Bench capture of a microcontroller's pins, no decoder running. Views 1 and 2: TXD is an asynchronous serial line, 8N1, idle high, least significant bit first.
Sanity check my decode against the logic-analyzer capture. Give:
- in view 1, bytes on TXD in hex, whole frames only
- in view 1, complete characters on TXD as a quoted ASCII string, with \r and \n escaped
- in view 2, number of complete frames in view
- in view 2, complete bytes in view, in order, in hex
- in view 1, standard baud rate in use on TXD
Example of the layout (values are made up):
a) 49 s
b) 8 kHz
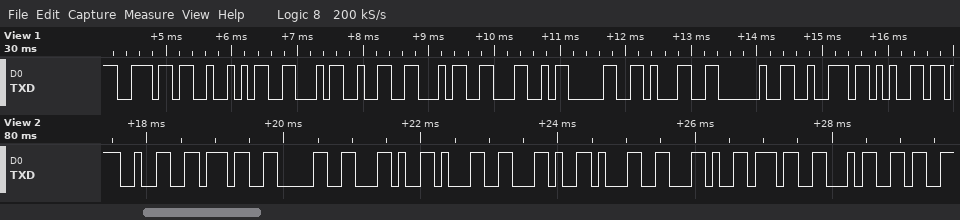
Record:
a) 0x6E 0x52 0x46 0x32 0x34 0x4C 0x30 0x31 0x20 0x72 0x65
b) "nRF24L01 re"
c) 10
d) 0x32 0x37 0x30 0x2C 0x31 0x2C 0x31 0x2C 0x37 0x34
e) 9600 baud
